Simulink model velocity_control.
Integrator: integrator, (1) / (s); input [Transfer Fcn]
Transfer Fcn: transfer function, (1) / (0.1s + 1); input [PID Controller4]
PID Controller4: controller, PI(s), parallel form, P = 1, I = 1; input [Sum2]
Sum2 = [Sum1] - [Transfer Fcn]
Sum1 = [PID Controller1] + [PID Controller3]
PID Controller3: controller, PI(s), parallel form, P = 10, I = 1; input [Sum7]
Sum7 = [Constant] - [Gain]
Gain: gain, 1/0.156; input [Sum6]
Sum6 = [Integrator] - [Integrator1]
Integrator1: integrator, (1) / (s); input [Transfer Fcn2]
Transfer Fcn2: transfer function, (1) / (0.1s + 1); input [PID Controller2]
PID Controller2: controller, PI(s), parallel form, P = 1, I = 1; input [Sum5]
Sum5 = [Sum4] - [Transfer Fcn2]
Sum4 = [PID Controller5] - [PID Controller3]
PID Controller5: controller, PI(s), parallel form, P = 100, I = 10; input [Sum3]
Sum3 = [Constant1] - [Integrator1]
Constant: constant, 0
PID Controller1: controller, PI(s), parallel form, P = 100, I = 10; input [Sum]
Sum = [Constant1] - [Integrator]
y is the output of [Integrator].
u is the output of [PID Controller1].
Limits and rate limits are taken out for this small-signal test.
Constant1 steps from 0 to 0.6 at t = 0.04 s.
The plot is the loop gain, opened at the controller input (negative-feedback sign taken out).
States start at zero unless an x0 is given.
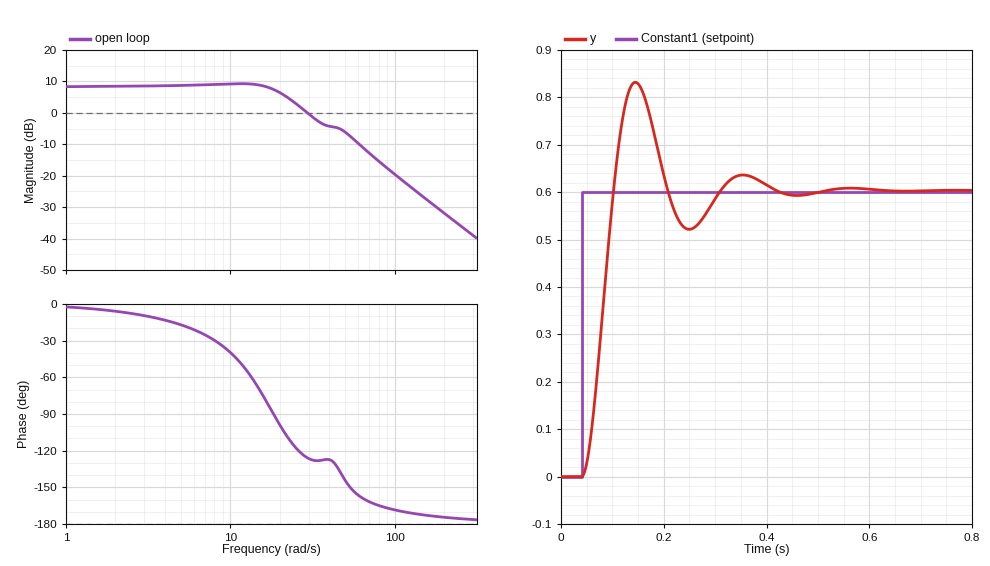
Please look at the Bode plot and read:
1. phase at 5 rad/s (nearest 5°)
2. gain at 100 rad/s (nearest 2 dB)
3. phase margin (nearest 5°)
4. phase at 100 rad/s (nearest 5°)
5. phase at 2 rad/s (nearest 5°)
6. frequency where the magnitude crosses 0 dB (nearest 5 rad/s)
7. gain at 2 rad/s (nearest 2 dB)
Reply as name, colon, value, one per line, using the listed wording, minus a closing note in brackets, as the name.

phase at 5 rad/s: -15°
gain at 100 rad/s: -20 dB
phase margin: 55°
phase at 100 rad/s: -170°
phase at 2 rad/s: -5°
frequency where the magnitude crosses 0 dB: 30 rad/s
gain at 2 rad/s: 8 dB
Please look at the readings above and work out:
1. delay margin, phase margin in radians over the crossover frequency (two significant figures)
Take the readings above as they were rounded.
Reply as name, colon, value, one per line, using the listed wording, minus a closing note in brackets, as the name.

delay margin, phase margin in radians over the crossover frequency: 0.032 s
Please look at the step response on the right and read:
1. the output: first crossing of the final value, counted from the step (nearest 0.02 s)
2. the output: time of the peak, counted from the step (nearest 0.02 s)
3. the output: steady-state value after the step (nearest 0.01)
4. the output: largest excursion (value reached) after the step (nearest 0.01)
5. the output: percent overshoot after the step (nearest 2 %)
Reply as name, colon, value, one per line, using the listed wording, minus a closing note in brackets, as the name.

the output: first crossing of the final value, counted from the step: 0.06 s
the output: time of the peak, counted from the step: 0.10 s
the output: steady-state value after the step: 0.60
the output: largest excursion (value reached) after the step: 0.83
the output: percent overshoot after the step: 38 %
